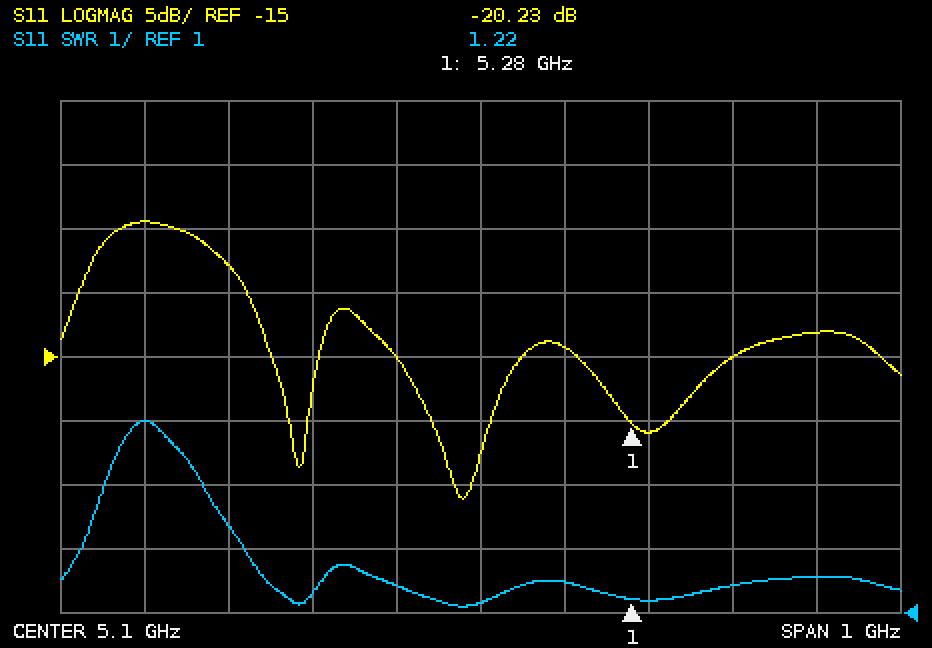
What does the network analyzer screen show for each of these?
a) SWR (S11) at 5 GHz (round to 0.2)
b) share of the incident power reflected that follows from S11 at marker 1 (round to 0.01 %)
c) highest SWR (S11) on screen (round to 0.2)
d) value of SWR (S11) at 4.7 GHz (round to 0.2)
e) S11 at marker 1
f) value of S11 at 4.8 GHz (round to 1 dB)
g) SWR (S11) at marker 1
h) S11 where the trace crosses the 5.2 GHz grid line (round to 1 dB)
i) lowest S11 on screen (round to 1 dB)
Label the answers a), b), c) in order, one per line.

a) 1.4
b) 0.95 %
c) 4.0
d) 4.0
e) -20.23 dB
f) -8 dB
g) 1.22
h) -14 dB
i) -26 dB
